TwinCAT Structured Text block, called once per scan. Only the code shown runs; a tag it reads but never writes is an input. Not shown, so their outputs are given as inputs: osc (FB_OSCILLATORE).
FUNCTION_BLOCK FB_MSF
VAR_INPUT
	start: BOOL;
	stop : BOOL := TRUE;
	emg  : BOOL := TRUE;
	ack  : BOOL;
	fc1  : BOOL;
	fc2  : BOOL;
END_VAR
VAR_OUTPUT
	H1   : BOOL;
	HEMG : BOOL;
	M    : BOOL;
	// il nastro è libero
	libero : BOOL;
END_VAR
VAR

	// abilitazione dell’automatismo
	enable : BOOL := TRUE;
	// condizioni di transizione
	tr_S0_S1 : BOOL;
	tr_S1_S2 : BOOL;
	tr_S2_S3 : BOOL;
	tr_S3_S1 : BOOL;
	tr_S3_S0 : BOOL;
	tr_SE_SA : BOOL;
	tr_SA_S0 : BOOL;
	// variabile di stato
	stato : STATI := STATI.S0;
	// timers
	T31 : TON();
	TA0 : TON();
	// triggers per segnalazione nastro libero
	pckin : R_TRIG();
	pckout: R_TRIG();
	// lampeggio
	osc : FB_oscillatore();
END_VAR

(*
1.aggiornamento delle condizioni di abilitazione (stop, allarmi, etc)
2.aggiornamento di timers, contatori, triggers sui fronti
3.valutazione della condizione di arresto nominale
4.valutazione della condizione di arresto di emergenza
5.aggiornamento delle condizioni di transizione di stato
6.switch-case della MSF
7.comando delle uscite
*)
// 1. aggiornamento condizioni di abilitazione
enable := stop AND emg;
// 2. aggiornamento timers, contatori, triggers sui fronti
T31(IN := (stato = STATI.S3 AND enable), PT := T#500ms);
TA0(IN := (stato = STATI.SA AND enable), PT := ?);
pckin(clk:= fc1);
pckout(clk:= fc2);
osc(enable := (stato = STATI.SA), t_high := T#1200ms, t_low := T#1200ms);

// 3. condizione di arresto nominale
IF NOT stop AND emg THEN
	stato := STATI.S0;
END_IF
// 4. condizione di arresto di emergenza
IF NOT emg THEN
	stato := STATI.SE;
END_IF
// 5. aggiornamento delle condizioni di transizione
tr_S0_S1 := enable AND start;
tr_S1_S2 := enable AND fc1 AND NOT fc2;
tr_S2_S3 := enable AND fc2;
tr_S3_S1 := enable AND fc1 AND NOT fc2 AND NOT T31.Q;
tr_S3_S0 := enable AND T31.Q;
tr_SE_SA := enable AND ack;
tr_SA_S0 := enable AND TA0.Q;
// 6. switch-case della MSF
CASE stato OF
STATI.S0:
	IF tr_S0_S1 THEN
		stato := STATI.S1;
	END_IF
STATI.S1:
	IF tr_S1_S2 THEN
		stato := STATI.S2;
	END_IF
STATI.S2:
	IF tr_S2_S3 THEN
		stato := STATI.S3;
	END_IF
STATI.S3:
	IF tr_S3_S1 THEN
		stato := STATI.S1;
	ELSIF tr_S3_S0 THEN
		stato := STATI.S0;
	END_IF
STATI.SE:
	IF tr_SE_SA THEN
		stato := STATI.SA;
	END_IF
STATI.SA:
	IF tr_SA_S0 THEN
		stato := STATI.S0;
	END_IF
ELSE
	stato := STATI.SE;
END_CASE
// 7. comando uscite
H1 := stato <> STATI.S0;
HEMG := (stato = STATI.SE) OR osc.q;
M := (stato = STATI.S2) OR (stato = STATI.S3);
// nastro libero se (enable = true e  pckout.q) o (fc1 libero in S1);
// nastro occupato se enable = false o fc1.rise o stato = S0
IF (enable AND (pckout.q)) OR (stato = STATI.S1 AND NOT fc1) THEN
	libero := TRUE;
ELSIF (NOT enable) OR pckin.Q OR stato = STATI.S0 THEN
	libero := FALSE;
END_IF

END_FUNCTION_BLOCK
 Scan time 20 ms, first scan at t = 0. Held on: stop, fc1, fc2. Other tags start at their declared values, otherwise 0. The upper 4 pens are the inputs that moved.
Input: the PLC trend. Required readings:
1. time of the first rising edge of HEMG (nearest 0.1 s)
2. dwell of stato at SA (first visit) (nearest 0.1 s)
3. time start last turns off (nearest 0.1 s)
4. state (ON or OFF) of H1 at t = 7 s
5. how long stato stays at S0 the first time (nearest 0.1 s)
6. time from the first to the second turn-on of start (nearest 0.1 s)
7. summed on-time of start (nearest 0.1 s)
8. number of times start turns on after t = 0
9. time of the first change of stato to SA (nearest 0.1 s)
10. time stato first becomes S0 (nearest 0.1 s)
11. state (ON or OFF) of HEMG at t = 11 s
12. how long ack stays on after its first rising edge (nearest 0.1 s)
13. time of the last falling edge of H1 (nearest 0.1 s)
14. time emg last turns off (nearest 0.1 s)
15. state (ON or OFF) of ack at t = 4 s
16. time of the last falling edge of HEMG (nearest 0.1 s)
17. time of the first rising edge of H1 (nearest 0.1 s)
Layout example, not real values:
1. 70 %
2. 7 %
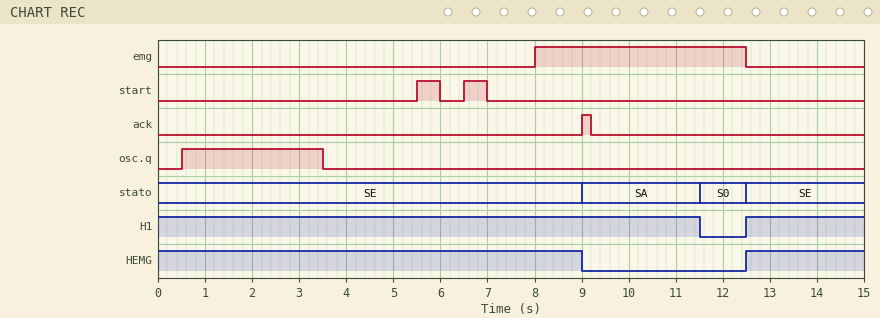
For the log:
1. 12.5 s
2. 2.5 s
3. 7.0 s
4. ON
5. 1.0 s
6. 1.0 s
7. 1.0 s
8. 2
9. 9.0 s
10. 11.5 s
11. OFF
12. 0.2 s
13. 11.5 s
14. 12.5 s
15. OFF
16. 9.0 s
17. 12.5 s
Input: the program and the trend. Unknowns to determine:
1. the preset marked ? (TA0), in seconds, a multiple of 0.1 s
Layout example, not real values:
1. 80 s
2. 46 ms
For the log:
1. 2.5 s
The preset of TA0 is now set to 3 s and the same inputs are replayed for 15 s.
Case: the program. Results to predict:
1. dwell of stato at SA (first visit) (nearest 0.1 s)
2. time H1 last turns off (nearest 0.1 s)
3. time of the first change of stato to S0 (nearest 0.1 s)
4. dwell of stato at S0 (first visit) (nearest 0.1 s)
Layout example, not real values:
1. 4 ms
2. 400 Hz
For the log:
1. 3.0 s
2. 12.0 s
3. 12.0 s
4. 0.5 s
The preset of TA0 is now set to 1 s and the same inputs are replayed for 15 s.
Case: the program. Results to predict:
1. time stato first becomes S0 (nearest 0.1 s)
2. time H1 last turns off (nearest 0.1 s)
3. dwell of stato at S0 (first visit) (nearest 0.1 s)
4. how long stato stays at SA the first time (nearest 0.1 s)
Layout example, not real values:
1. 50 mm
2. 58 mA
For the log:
1. 10.0 s
2. 10.0 s
3. 2.5 s
4. 1.0 s
